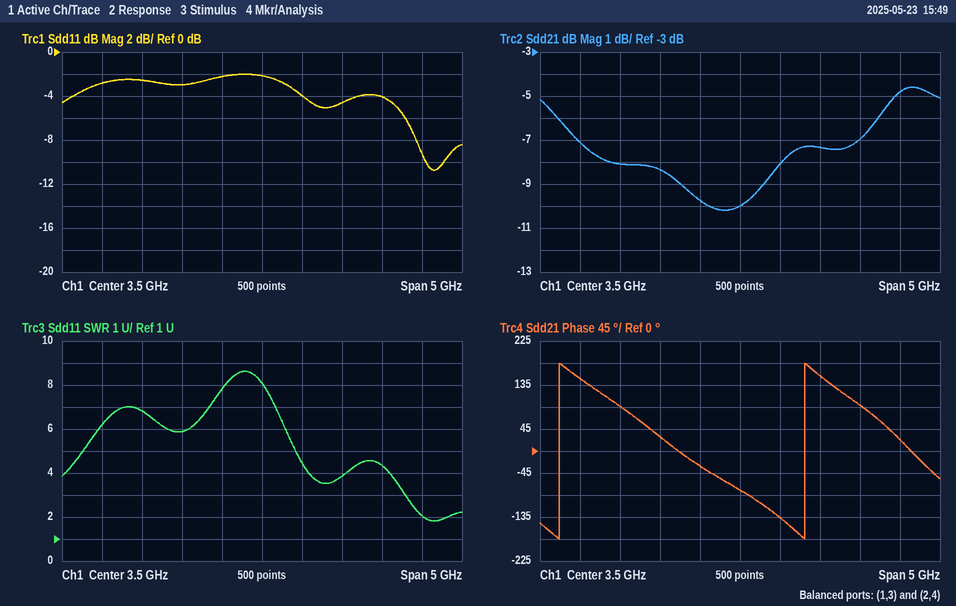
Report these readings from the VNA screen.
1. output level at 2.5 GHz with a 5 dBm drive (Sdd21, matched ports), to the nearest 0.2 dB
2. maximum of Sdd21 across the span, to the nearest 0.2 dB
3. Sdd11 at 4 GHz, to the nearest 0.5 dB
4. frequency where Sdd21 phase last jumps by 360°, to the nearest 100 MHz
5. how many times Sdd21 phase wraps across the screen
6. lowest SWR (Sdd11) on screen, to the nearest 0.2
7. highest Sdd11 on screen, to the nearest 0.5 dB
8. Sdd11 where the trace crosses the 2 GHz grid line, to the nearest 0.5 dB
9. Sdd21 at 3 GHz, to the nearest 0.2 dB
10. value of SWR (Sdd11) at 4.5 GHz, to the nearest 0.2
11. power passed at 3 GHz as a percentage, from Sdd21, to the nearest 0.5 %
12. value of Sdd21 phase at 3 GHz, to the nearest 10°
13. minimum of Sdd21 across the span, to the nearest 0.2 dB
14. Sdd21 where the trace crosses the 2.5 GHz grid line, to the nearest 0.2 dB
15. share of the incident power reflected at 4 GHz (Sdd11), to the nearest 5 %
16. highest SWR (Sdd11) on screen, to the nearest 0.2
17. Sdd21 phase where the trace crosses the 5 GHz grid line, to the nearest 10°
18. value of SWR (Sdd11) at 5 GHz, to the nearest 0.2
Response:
-3.4 dBm
-4.6 dB
-4.0 dB
4.3 GHz
2
1.8
-2.0 dB
-2.5 dB
-9.8 dB
3.8
10.5 %
-30°
-10.2 dB
-8.4 dB
40 %
8.6
90°
4.4
